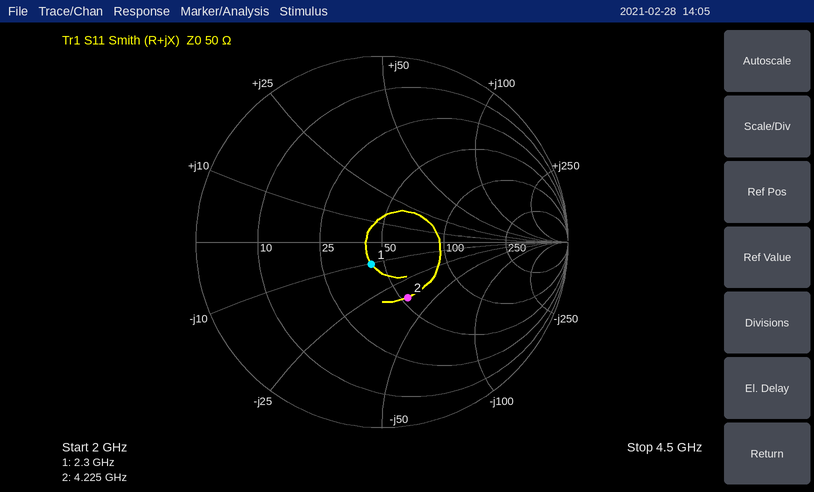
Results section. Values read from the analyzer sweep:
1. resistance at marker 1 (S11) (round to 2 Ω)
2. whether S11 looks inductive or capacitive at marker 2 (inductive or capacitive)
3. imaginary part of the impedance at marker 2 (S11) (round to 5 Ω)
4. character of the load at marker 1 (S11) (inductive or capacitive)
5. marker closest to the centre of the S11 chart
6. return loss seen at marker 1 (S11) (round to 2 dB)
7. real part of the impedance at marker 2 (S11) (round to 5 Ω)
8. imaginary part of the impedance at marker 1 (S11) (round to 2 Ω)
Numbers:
44 Ω
capacitive
-35 Ω
capacitive
marker 1
18 dB
55 Ω
-10 Ω
